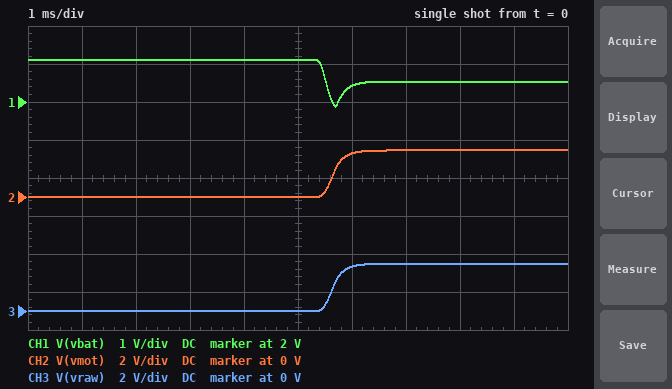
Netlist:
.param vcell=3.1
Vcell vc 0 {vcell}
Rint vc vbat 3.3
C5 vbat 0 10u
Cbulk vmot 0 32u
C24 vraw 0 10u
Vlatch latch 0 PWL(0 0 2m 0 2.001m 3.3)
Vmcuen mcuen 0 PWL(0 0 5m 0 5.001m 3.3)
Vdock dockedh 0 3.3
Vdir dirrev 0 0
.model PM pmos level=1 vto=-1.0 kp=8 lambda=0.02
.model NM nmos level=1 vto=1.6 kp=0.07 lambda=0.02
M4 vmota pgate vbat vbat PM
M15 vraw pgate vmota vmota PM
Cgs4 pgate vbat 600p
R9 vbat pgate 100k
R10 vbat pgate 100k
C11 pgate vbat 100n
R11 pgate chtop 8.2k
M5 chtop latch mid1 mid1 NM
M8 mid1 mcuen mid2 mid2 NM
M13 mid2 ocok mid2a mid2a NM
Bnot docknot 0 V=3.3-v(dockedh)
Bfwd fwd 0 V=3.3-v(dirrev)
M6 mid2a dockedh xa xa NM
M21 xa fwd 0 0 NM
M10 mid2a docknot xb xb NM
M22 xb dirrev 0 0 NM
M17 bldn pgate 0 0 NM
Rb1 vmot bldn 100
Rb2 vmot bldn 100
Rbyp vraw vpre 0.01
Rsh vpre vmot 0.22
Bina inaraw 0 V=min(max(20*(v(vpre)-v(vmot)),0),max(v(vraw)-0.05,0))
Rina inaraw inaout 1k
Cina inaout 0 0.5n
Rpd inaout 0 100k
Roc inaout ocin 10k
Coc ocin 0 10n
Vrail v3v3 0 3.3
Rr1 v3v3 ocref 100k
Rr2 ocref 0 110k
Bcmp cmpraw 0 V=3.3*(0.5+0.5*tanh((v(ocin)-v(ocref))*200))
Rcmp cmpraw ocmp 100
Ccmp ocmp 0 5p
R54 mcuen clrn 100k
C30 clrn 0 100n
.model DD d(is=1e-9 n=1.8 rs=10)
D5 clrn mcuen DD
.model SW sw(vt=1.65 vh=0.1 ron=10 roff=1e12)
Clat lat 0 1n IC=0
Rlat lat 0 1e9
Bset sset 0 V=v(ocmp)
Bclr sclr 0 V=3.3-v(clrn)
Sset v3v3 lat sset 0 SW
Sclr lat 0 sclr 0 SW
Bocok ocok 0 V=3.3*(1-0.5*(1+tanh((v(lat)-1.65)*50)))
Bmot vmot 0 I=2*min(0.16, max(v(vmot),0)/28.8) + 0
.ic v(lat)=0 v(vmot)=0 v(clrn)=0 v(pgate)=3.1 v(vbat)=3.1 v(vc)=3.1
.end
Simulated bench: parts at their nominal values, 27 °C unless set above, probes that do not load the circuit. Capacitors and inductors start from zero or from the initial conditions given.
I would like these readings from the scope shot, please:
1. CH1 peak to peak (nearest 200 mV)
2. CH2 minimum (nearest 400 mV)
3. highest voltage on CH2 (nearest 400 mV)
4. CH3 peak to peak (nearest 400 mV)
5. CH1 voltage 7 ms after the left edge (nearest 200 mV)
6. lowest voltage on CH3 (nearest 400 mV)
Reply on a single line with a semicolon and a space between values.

1.2 V; 0 V; 2.4 V; 2.4 V; 2.6 V; 0 V
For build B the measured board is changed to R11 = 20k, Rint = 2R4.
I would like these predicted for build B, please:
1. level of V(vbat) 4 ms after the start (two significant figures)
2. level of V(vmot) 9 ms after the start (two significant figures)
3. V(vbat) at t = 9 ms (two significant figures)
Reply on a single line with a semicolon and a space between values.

3.1 V; 2.6 V; 2.7 V
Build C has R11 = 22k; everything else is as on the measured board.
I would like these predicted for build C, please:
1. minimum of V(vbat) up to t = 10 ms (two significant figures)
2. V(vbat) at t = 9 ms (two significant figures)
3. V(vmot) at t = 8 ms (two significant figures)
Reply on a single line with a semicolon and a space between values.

2.2 V; 2.5 V; 2.4 V
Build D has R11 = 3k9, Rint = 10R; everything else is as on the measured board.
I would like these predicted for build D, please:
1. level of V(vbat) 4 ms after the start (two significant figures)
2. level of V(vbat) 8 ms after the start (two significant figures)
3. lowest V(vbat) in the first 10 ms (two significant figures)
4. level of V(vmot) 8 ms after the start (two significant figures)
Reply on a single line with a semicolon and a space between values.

3.1 V; 1.9 V; 1.0 V; 1.8 V
